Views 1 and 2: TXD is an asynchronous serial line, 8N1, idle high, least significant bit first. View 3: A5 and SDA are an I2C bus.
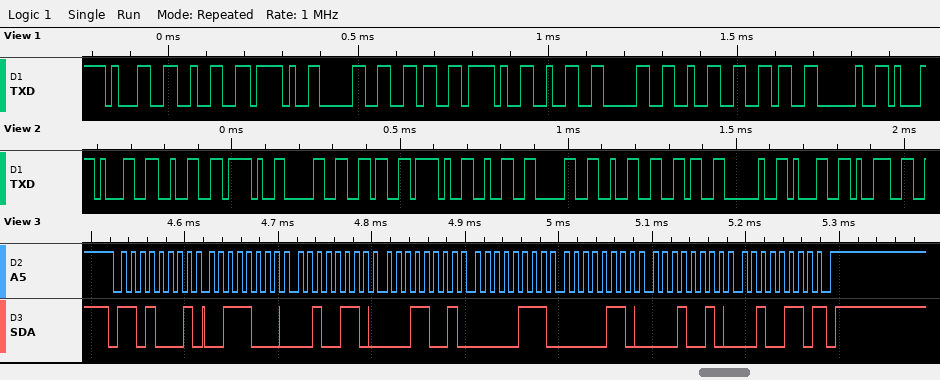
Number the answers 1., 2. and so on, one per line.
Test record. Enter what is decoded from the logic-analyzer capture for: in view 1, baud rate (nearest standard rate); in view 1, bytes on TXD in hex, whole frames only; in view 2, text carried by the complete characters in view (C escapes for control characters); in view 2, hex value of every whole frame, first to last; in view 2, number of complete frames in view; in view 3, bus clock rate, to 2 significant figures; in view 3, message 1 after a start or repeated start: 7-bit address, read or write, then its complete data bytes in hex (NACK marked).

1. 57600 baud
2. 31 32 2F 30 36 2F 32 30 32 36 20
3. "12/06/2026 19"
4. 0x31 0x32 0x2F 0x30 0x36 0x2F 0x32 0x30 0x32 0x36 0x20 0x31 0x39
5. 13
6. 100 kHz
7. 0x68 read: 38 26 19 07 06 12 26 NACK
